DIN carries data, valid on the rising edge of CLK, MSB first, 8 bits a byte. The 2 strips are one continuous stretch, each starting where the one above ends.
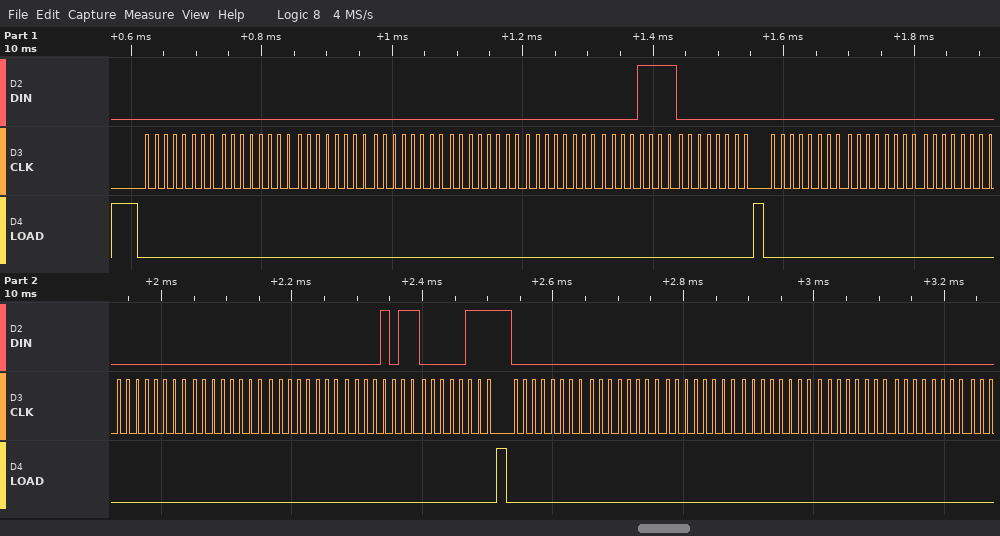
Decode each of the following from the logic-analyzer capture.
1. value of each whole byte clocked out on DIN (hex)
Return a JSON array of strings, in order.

["00 00 00 00 00 00 0F 00 00 00 00 00 00 00 0B 07 00 00 00 00 00 00"]
